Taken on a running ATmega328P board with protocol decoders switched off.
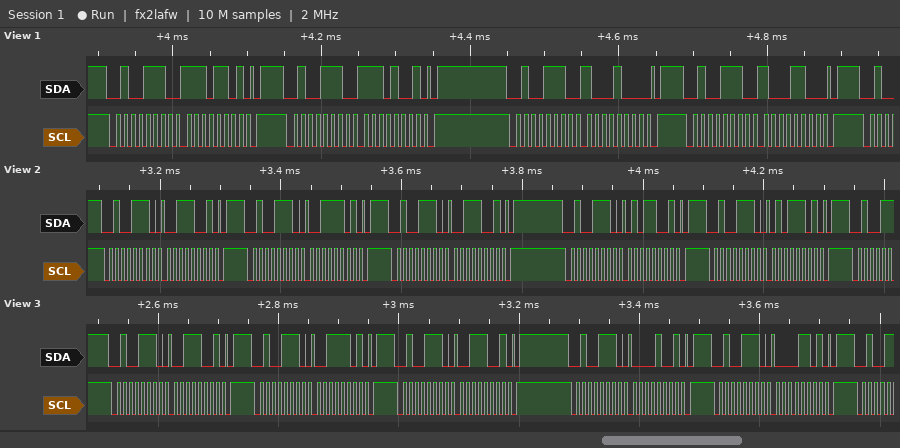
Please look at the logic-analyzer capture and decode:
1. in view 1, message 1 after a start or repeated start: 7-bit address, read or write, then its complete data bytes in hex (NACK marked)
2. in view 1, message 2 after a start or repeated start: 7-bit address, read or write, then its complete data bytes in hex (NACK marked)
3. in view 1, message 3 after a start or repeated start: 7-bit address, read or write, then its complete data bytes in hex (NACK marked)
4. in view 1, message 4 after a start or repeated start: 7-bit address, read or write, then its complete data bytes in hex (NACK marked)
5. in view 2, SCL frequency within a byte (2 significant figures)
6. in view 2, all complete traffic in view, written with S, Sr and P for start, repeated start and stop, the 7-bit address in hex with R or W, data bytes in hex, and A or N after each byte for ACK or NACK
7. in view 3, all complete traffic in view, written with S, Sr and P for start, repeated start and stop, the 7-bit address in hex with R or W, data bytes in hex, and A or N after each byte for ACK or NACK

0x27 write: ED
0x27 write: E9
0x27 write: 88
0x27 write: 8C
100 kHz
S 27W A 39 A P S 27W A 3D A P S 27W A 39 A P S 27W A 59 A P S 27W A 5D A P
S 27W A 39 A P S 27W A 3D A P S 27W A 39 A P S 27W A 09 A P S 27W A 0D A P
